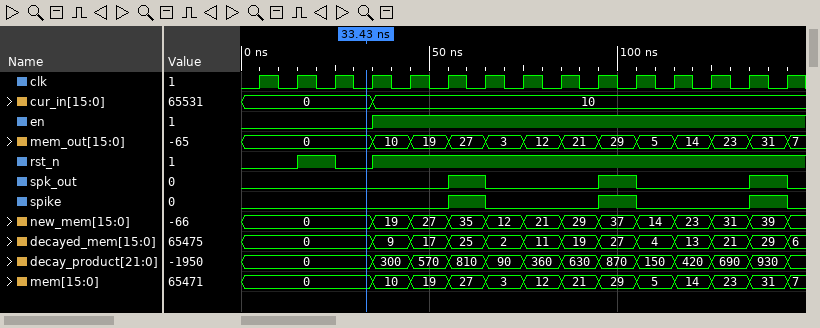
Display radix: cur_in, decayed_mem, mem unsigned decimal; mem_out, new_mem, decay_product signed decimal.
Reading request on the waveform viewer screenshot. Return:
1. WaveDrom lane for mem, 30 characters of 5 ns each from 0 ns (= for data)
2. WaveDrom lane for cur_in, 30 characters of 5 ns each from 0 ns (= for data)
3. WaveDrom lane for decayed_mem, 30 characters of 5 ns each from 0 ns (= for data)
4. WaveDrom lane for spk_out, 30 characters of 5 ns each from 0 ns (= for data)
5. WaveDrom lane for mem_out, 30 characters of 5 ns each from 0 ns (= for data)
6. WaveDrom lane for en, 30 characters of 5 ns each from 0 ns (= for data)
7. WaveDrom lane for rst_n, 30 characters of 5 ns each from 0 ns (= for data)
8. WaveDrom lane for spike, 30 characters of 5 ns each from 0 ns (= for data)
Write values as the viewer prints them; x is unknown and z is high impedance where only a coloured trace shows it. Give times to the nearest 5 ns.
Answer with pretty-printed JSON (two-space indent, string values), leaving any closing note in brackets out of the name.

{
  "WaveDrom lane for mem, 30 characters of 5 ns each from 0 ns": "{name: 'mem', wave: '=......=.=.=.=.=.=.=.=.=.=.=.=', data: '0 10 19 27 3 12 21 29 5 14 23 31 7'}",
  "WaveDrom lane for cur_in, 30 characters of 5 ns each from 0 ns": "{name: 'cur_in', wave: '=......=......................', data: '0 10'}",
  "WaveDrom lane for decayed_mem, 30 characters of 5 ns each from 0 ns": "{name: 'decayed_mem', wave: '=......=.=.=.=.=.=.=.=.=.=.=.=', data: '0 9 17 25 2 11 19 27 4 13 21 29 6'}",
  "WaveDrom lane for spk_out, 30 characters of 5 ns each from 0 ns": "{name: 'spk_out', wave: '0..........1.0.....1.0.....1.0'}",
  "WaveDrom lane for mem_out, 30 characters of 5 ns each from 0 ns": "{name: 'mem_out', wave: '=......=.=.=.=.=.=.=.=.=.=.=.=', data: '0 10 19 27 3 12 21 29 5 14 23 31 7'}",
  "WaveDrom lane for en, 30 characters of 5 ns each from 0 ns": "{name: 'en', wave: '0......1......................'}",
  "WaveDrom lane for rst_n, 30 characters of 5 ns each from 0 ns": "{name: 'rst_n', wave: '0..1.0.1......................'}",
  "WaveDrom lane for spike, 30 characters of 5 ns each from 0 ns": "{name: 'spike', wave: '0..........1.0.....1.0.....1.0'}"
}
